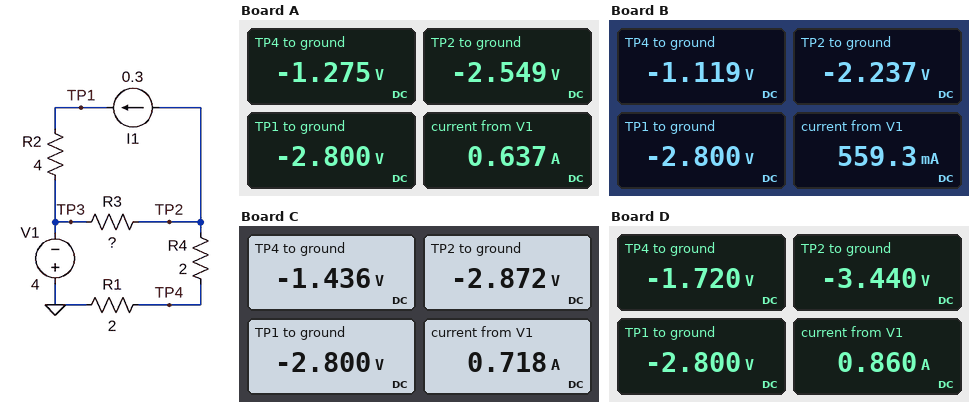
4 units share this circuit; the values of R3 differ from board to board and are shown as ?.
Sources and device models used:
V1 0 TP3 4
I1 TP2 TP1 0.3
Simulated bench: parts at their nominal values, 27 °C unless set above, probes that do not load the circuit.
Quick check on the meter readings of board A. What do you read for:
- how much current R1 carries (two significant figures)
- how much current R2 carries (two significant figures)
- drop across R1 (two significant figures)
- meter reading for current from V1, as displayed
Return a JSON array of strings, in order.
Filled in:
["640 mA", "300 mA", "1.3 V", "0.637 A"]
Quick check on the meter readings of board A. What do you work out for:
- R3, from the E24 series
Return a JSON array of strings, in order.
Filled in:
["4.3 Ω"]
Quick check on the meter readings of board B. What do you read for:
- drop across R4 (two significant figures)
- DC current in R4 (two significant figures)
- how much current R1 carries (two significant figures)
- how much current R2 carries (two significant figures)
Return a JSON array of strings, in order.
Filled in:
["1.1 V", "560 mA", "560 mA", "300 mA"]
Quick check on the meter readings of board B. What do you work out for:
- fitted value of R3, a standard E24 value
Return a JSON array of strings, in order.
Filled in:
["6.8 Ω"]
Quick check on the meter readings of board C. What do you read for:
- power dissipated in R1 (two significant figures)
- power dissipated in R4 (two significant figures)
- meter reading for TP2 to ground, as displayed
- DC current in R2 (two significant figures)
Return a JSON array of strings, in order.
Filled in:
["1.0 W", "1.0 W", "-2.872 V", "300 mA"]
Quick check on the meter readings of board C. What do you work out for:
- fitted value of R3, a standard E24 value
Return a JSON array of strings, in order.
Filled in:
["2.7 Ω"]
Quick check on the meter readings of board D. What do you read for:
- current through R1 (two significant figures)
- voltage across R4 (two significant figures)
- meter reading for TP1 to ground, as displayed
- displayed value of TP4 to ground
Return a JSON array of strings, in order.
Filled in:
["860 mA", "1.7 V", "-2.800 V", "-1.720 V"]
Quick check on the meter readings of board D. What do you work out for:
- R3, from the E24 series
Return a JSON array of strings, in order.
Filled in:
["1 Ω"]
